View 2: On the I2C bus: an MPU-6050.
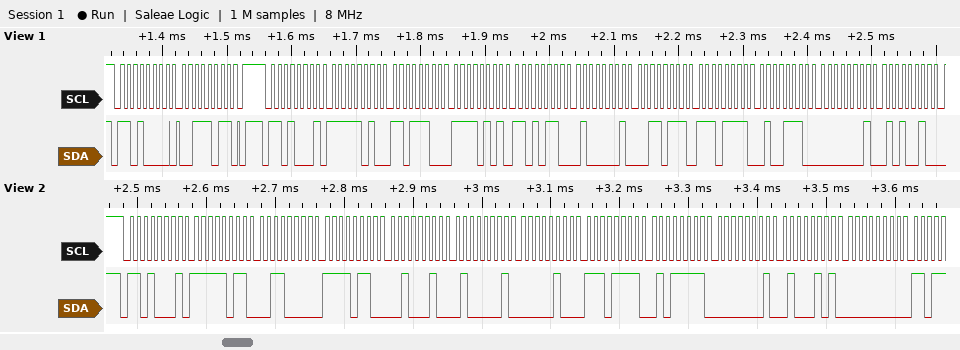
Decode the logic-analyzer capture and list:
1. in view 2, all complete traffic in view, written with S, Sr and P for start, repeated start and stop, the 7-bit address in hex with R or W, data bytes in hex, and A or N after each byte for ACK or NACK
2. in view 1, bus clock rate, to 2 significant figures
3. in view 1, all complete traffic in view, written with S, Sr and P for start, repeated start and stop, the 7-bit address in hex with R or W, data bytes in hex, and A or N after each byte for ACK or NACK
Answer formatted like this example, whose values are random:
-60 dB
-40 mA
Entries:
S 68R A FB A 30 A F6 A 22 A 41 A 04 A EF A 5F A 01 A 45 A 00 A
100 kHz
S 68W A 3B A P S 68R A FA A DC A F5 A D6 A 41 A 37 A EF A 4E A 01 A 52 A
